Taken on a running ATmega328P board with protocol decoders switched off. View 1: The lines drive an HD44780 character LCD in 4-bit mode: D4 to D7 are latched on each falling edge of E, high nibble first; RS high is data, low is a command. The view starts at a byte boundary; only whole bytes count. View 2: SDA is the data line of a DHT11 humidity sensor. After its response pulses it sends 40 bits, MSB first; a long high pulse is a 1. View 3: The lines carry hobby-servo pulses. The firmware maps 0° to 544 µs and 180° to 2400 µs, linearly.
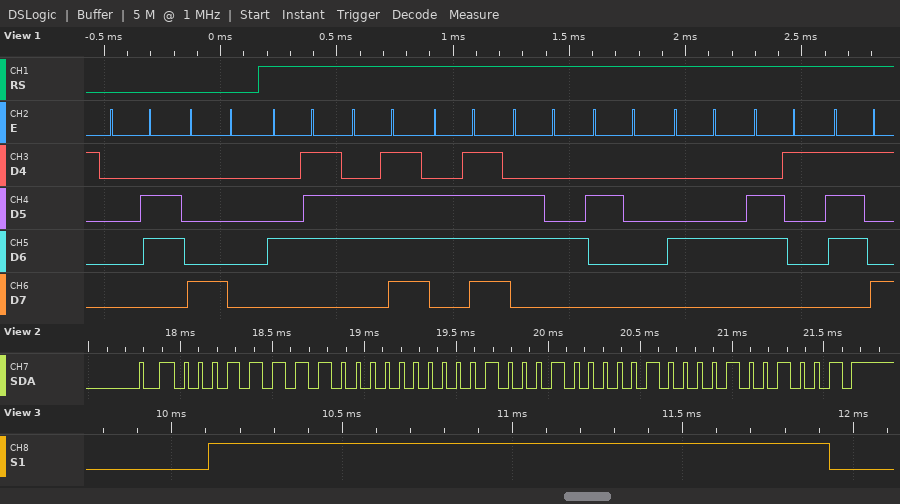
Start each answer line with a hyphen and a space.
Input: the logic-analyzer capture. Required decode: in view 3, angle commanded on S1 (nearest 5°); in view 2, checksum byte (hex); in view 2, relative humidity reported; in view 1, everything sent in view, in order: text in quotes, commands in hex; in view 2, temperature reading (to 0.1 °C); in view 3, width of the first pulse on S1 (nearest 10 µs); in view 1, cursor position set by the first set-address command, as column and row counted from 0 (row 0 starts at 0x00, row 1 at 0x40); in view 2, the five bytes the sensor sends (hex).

- 125°
- 0x49
- 31 %
- 0x06 0x80 "Good Day"
- 34.8 °C
- 1820 µs
- column 0, row 0
- 1F 00 22 08 49
